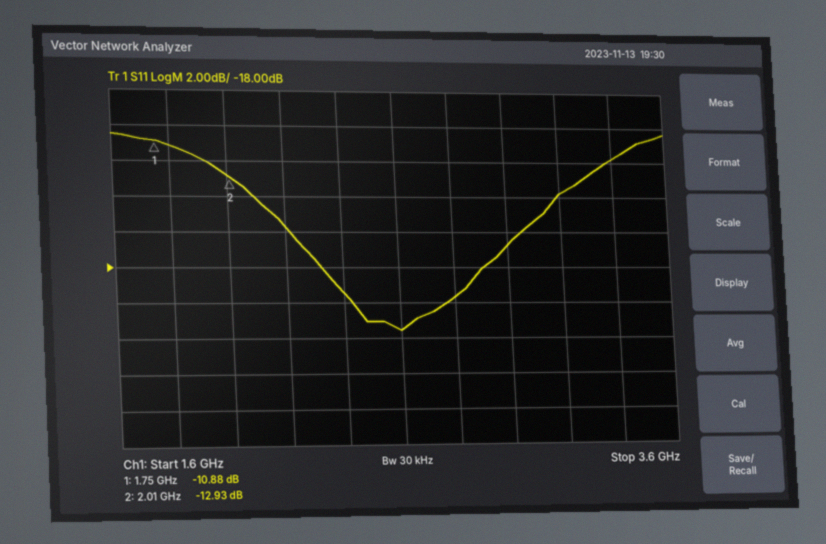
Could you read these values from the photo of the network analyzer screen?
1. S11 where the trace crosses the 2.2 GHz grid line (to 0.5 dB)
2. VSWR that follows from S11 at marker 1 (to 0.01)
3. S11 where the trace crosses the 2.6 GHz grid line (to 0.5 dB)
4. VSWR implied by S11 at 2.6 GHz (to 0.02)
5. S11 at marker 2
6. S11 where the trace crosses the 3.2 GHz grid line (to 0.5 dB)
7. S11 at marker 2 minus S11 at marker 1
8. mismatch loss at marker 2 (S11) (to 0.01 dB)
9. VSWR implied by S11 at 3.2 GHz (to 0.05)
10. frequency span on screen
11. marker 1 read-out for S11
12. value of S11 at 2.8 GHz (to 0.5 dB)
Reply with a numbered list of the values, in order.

1. -15.5 dB
2. 1.80
3. -21.5 dB
4. 1.18
5. -12.93 dB
6. -14.0 dB
7. -2.05 dB
8. 0.23 dB
9. 1.50
10. 2 GHz
11. -10.88 dB
12. -19.5 dB
